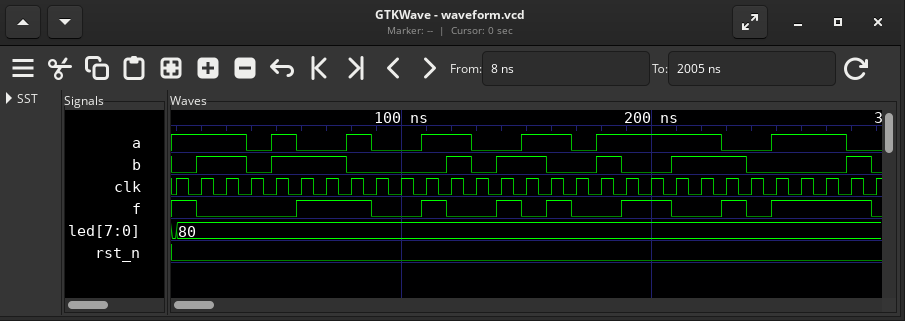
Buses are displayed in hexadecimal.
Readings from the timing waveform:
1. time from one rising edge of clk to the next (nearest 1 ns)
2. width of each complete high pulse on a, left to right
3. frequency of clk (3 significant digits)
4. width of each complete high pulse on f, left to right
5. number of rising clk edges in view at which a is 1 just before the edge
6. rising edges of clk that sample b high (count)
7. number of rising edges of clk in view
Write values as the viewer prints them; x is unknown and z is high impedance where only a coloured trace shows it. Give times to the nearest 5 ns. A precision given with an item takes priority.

10 ns
10 ns, 10 ns, 20 ns, 20 ns, 50 ns, 30 ns
100 MHz
30 ns, 10 ns, 10 ns, 10 ns, 20 ns, 10 ns, 40 ns
17
13
29
